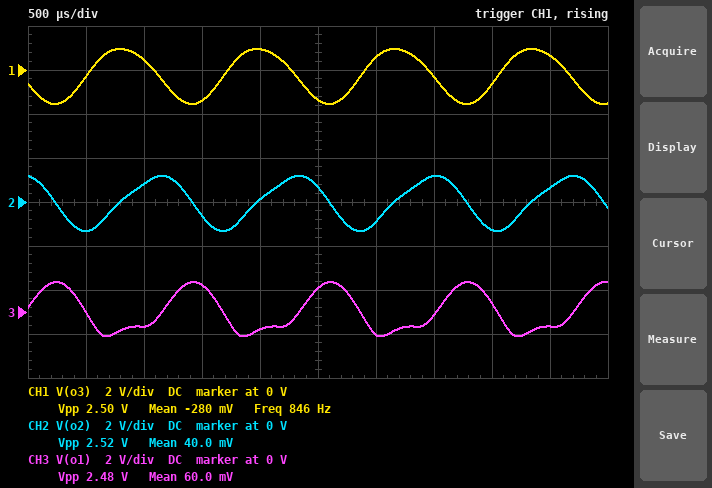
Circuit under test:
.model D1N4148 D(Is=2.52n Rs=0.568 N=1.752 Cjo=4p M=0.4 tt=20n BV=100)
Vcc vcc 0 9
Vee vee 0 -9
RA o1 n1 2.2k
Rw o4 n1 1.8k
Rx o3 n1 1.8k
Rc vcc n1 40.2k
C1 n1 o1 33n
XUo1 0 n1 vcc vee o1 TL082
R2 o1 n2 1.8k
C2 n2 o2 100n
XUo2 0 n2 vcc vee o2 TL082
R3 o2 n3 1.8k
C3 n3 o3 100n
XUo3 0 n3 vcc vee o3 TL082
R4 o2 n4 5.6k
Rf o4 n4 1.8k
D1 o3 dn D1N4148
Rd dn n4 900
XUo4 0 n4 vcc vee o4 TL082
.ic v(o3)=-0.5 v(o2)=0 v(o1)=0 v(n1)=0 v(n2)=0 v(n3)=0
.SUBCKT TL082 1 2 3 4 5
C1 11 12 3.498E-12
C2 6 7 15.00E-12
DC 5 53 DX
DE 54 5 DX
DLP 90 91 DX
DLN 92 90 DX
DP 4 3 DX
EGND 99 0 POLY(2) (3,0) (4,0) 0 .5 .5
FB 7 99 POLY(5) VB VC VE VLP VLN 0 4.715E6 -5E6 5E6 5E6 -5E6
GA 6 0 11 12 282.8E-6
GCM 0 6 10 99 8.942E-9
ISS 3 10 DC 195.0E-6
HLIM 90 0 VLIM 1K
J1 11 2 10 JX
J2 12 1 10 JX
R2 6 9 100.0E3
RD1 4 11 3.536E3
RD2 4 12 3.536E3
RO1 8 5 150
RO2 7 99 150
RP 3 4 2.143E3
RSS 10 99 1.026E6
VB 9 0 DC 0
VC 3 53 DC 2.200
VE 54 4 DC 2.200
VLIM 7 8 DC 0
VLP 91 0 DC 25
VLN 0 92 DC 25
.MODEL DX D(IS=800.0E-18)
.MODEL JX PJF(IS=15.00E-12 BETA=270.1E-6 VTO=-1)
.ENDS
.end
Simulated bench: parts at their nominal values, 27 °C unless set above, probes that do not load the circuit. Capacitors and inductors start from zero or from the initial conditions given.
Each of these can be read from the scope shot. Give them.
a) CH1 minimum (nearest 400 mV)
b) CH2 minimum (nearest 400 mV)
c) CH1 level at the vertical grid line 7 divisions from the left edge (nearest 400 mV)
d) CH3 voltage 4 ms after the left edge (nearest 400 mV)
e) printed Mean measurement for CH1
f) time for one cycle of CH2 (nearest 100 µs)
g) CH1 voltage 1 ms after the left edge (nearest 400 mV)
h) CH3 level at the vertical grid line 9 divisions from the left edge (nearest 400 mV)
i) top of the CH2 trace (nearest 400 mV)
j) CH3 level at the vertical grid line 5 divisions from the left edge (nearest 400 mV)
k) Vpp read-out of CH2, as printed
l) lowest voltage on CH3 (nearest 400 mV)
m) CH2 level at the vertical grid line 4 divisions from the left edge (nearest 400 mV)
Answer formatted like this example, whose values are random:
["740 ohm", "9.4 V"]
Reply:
["-1.6 V", "-1.2 V", "-400 mV", "400 mV", "-280 mV", "1.2 ms", "400 mV", "-800 mV", "1.2 V", "1.2 V", "2.52 V", "-1.2 V", "0 V"]
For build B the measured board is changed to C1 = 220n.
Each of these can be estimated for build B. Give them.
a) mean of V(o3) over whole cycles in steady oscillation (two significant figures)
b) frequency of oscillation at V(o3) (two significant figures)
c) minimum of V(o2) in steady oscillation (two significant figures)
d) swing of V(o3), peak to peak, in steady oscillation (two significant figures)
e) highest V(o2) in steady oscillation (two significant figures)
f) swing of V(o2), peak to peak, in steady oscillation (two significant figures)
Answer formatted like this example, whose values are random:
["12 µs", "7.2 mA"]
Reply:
["7.1 V", "240 Hz", "-5.2 V", "2.9 V", "1.1 V", "6.3 V"]
